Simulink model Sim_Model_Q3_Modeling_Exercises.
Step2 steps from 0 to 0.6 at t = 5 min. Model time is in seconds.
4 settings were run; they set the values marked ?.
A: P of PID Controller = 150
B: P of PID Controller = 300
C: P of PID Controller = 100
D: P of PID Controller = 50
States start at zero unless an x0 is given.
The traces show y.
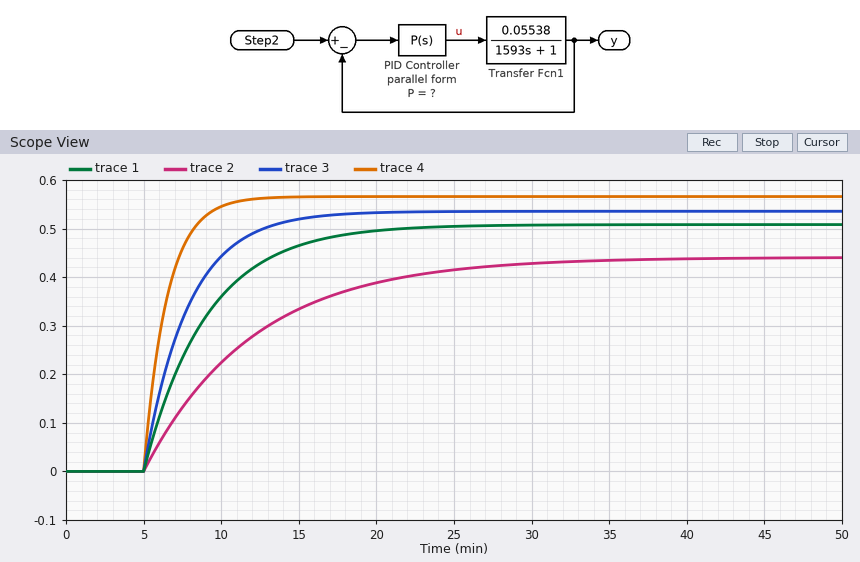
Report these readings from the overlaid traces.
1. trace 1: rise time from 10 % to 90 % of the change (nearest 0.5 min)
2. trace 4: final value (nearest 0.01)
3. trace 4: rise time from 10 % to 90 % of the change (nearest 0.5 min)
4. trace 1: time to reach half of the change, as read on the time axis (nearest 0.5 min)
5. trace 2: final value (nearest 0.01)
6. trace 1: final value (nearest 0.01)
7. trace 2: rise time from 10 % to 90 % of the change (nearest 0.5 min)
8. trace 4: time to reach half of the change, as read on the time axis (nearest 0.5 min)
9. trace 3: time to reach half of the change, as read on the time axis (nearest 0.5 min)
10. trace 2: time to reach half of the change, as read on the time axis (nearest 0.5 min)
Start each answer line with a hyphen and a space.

- 9.0 min
- 0.57
- 3.5 min
- 8.0 min
- 0.44
- 0.51
- 15.5 min
- 6.0 min
- 7.0 min
- 10.0 min
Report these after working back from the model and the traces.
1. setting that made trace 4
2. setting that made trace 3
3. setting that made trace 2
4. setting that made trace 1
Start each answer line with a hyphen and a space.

- B
- A
- D
- C
